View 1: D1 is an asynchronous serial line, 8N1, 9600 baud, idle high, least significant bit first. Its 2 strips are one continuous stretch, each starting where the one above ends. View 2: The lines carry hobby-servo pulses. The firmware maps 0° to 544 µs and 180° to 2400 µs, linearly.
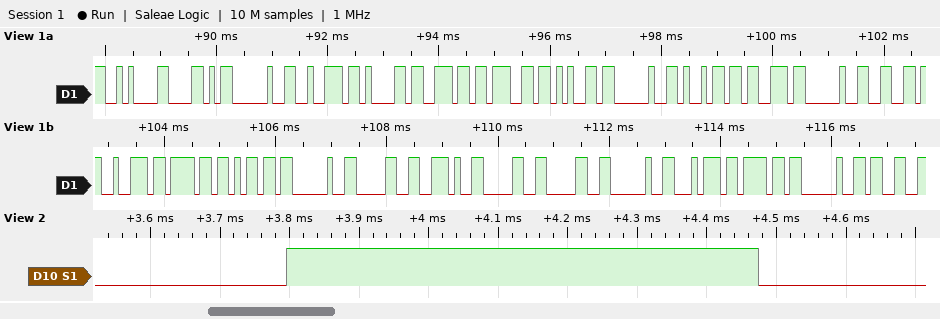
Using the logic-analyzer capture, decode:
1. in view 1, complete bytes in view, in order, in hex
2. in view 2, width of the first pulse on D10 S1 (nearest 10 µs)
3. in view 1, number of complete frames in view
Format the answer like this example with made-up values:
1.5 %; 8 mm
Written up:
0A 58 20 72 61 6E 67 65 20 69 73 20 66 72 6F 6D 20 30 2E 30 30 20 74 6F 20 33; 680 µs; 26
